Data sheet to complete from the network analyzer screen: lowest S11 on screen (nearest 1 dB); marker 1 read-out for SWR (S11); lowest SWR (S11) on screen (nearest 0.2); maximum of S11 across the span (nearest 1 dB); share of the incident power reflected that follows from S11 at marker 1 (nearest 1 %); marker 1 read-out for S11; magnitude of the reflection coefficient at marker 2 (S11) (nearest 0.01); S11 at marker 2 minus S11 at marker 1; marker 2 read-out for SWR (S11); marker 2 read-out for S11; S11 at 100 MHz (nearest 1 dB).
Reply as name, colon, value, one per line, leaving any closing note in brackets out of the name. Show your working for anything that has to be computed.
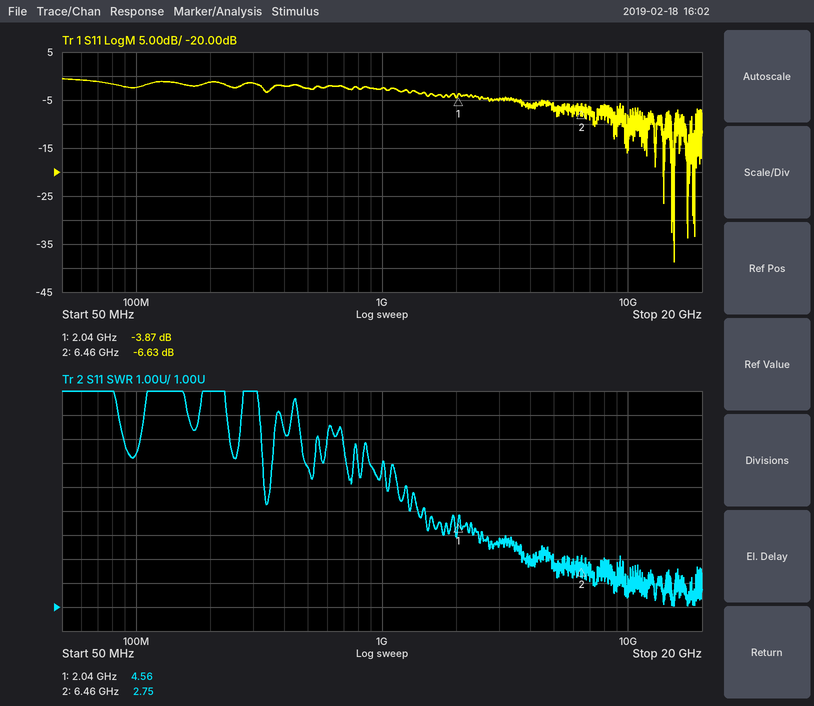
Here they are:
lowest S11 on screen: -39 dB
marker 1 read-out for SWR: 4.56
lowest SWR (S11) on screen: 1.0
maximum of S11 across the span: -1 dB
share of the incident power reflected that follows from S11 at marker 1: 10^(-3.87/10) ≈ 41 %
marker 1 read-out for S11: -3.87 dB
magnitude of the reflection coefficient at marker 2 (S11): 10^(-6.63/20) ≈ 0.47
S11 at marker 2 minus S11 at marker 1: -6.63 − (-3.87) = -2.76 dB
marker 2 read-out for SWR: 2.75
marker 2 read-out for S11: -6.63 dB
S11 at 100 MHz: -2 dB
